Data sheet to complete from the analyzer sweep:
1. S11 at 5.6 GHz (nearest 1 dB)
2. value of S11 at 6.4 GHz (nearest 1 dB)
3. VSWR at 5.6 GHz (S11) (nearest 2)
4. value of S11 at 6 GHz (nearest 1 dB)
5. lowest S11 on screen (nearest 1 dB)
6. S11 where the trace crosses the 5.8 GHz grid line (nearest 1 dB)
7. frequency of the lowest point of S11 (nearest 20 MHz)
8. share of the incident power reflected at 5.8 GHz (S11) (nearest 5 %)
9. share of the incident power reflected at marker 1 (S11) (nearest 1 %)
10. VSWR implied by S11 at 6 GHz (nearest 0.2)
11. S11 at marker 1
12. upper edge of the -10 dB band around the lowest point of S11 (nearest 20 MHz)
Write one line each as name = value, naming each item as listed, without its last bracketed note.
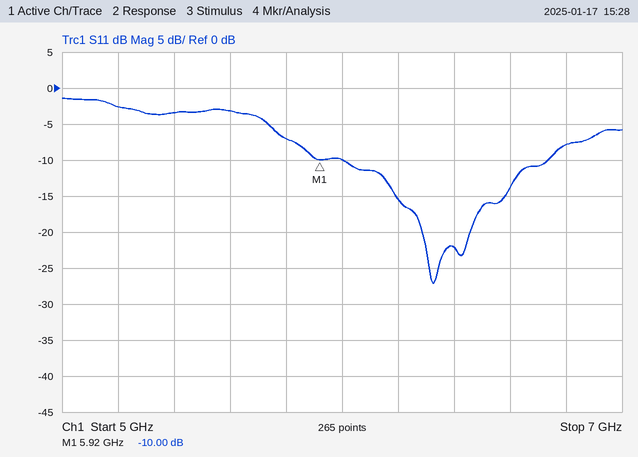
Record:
S11 at 5.6 GHz = -3 dB
value of S11 at 6.4 GHz = -22 dB
VSWR at 5.6 GHz (S11) = 6
value of S11 at 6 GHz = -10 dB
lowest S11 on screen = -27 dB
S11 where the trace crosses the 5.8 GHz grid line = -7 dB
frequency of the lowest point of S11 = 6.32 GHz
share of the incident power reflected at 5.8 GHz (S11) = 20 %
share of the incident power reflected at marker 1 (S11) = 10 %
VSWR implied by S11 at 6 GHz = 2.0
S11 at marker 1 = -10.00 dB
upper edge of the -10 dB band around the lowest point of S11 = 6.74 GHz
